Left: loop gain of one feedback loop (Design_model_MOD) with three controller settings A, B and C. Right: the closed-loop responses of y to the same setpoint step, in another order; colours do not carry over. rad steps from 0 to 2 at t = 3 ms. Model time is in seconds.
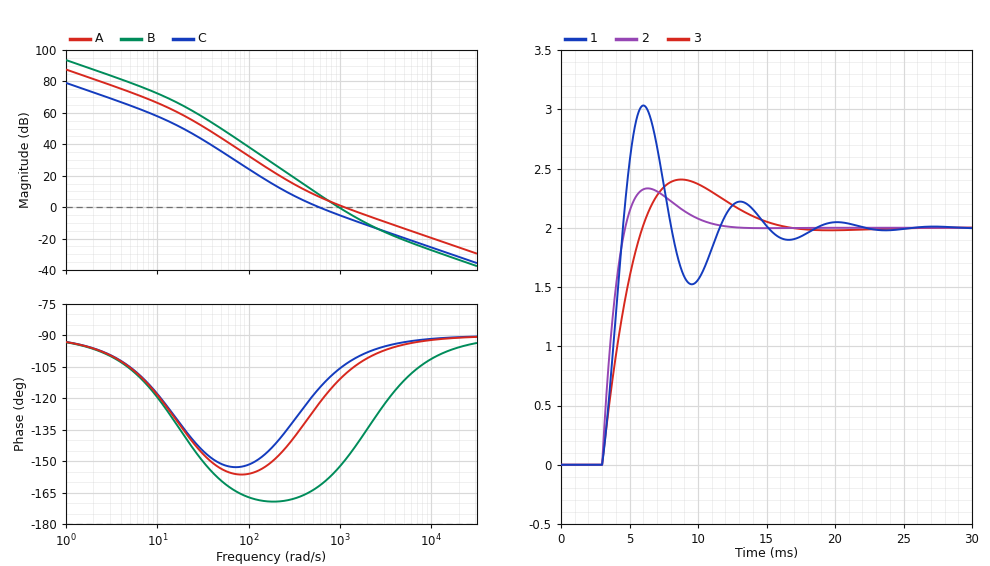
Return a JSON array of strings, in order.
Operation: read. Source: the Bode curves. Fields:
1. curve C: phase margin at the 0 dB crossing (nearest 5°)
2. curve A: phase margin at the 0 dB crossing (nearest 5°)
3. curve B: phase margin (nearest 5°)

["65°", "70°", "25°"]
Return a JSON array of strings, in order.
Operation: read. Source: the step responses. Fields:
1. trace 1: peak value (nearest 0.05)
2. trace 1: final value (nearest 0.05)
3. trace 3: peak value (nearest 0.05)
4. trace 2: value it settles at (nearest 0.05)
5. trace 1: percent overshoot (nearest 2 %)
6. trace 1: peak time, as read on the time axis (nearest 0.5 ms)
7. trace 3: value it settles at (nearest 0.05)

["3.05", "2.00", "2.40", "2.00", "52 %", "6.0 ms", "2.00"]
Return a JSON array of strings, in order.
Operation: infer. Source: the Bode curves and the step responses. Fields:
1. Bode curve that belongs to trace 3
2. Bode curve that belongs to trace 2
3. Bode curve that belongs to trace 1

["C", "A", "B"]
